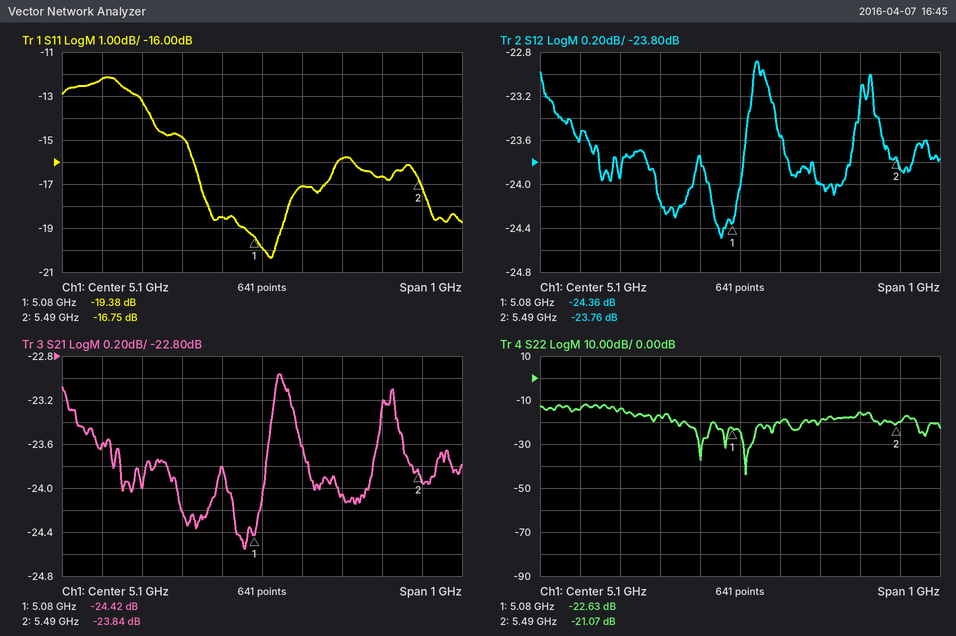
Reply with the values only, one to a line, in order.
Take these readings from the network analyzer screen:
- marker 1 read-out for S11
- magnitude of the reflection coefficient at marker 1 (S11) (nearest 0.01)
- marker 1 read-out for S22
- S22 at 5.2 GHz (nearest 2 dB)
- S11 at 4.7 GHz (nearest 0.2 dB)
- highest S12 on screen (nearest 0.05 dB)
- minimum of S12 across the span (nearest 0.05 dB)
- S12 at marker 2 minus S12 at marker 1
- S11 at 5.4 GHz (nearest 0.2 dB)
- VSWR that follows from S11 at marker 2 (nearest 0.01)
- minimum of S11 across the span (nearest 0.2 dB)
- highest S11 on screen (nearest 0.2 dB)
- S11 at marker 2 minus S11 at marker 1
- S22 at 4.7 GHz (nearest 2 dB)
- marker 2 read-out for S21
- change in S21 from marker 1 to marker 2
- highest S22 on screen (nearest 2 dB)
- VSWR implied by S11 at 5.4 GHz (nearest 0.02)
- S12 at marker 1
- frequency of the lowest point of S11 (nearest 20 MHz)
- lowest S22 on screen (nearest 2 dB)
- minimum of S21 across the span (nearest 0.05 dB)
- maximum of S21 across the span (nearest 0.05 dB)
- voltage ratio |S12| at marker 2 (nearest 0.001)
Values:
-19.38 dB
0.11
-22.63 dB
-20 dB
-12.2 dB
-22.90 dB
-24.50 dB
0.60 dB
-16.6 dB
1.34
-20.4 dB
-12.2 dB
2.63 dB
-14 dB
-23.84 dB
0.58 dB
-12 dB
1.34
-24.36 dB
5.12 GHz
-44 dB
-24.55 dB
-22.95 dB
0.065
